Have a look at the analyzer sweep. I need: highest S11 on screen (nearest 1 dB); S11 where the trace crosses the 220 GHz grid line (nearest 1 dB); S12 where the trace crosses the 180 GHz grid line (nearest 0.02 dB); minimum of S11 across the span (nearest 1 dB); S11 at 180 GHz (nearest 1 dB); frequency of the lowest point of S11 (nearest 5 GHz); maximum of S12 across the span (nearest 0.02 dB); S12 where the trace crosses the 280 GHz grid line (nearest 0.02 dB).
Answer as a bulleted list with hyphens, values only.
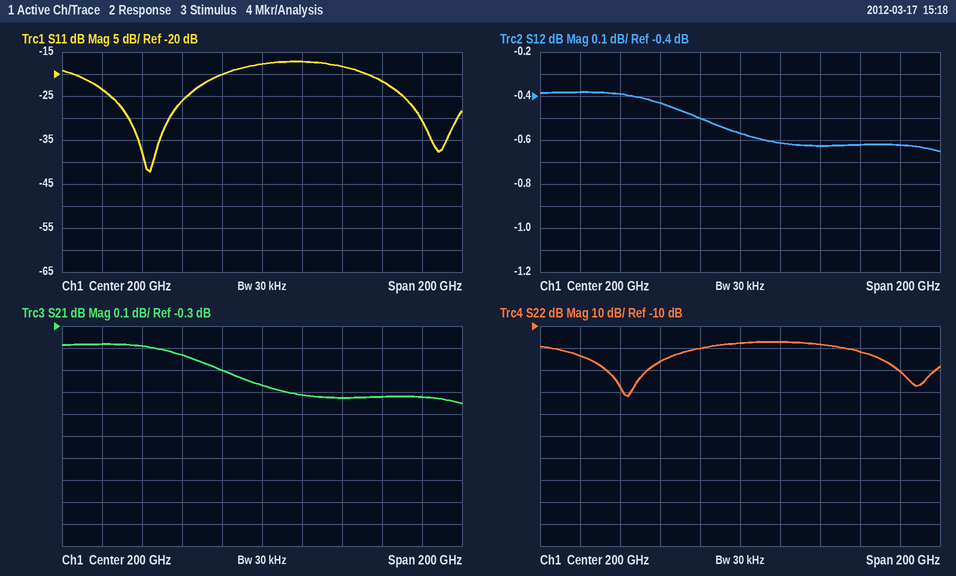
- -17 dB
- -17 dB
- -0.50 dB
- -42 dB
- -20 dB
- 145 GHz
- -0.38 dB
- -0.62 dB
